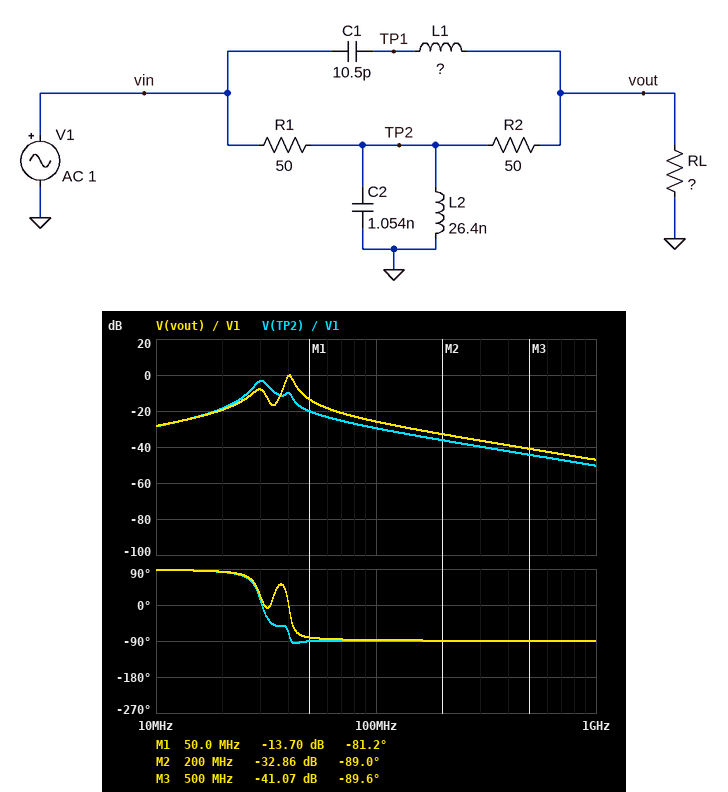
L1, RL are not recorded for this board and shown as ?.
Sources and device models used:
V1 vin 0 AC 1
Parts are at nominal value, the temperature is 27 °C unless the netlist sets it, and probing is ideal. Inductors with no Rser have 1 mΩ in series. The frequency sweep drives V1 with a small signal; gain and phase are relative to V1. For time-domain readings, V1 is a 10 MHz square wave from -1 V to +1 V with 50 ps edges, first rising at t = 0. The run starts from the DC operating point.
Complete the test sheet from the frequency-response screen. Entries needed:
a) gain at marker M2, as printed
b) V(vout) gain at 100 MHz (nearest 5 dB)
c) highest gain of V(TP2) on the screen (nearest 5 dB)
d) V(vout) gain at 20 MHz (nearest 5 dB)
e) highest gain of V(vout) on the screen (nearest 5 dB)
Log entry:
-32.86 dB
-25 dB
-5 dB
-20 dB
0 dB
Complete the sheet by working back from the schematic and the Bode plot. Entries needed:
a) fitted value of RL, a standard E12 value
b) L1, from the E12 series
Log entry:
56 Ω
1.5 µH
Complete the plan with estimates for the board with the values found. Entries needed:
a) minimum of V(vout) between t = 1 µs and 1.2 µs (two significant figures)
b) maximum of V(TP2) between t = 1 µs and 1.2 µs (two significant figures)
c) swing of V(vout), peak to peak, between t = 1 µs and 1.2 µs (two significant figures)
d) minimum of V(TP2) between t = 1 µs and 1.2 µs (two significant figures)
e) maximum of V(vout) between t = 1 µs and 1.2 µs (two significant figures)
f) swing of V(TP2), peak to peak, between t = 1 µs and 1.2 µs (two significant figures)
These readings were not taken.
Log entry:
-270 mV
360 mV
530 mV
-360 mV
270 mV
720 mV
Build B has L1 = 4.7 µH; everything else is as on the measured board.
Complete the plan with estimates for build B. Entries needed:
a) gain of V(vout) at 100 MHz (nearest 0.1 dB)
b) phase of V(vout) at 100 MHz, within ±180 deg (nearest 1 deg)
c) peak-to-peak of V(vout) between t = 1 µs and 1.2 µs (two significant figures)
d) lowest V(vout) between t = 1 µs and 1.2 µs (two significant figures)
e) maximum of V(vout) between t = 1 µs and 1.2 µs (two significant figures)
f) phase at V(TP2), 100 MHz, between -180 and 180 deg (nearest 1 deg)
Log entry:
-31.4 dB
-88 deg
440 mV
-220 mV
220 mV
-88 deg
